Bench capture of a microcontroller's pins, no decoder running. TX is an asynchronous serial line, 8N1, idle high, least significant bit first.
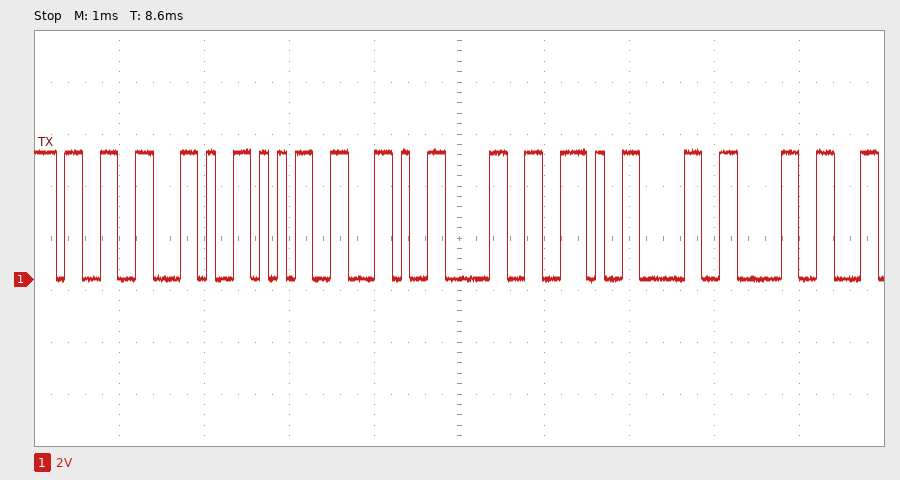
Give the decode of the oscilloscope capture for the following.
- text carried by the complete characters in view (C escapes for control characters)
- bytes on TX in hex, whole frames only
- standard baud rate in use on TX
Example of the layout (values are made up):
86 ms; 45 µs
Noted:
"3,5,0.00"; 0x33 0x2C 0x35 0x2C 0x30 0x2E 0x30 0x30; 9600 baud
